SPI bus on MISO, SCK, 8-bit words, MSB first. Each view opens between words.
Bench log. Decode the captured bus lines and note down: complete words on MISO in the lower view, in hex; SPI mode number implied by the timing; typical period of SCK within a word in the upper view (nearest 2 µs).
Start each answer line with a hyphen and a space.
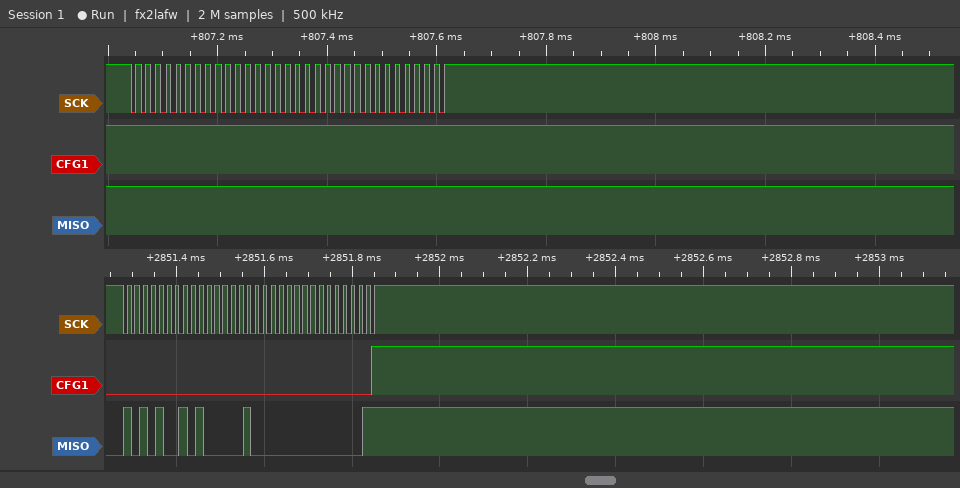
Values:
- A9, 41, 00, 03
- 3
- 18 µs
